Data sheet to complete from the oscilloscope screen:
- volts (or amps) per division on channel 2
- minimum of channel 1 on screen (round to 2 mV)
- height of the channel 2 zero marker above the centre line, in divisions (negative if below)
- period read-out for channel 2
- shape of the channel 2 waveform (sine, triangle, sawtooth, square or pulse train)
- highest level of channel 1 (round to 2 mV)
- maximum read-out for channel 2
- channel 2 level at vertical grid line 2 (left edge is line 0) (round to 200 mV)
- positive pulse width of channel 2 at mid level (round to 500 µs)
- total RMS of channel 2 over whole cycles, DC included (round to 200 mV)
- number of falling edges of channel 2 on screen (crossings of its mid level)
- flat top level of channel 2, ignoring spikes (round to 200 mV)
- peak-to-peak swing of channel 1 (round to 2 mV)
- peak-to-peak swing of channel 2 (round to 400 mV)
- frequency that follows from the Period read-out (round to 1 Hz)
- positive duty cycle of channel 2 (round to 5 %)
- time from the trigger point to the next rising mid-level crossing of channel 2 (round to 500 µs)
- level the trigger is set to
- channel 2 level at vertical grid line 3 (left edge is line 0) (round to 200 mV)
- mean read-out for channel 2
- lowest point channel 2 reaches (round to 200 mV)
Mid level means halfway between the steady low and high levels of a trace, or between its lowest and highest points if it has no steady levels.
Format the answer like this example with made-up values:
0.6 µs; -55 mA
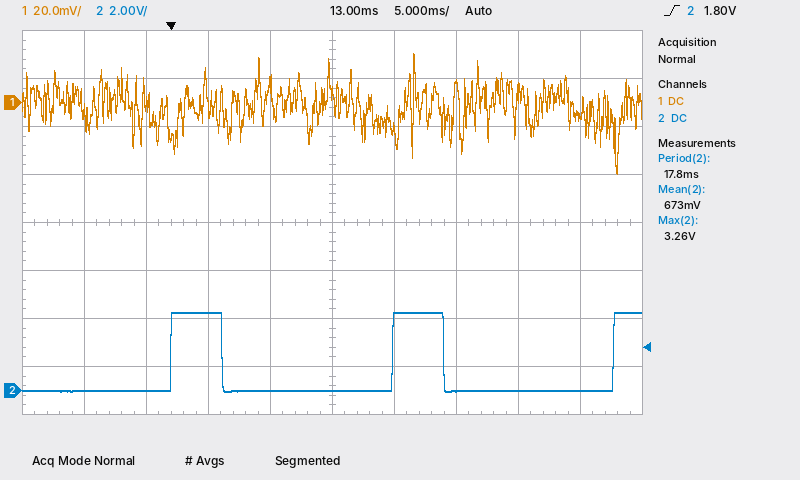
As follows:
2 V; -30 mV; -3.5 div; 17.8 ms; pulse train; 20 mV; 3.26 V; 0.0 V; 4.0 ms; 1.6 V; 2; 3.2 V; 50 mV; 3.2 V; 56 Hz; 25 %; 18.0 ms; 1.80 V; 3.2 V; 673 mV; 0.0 V
